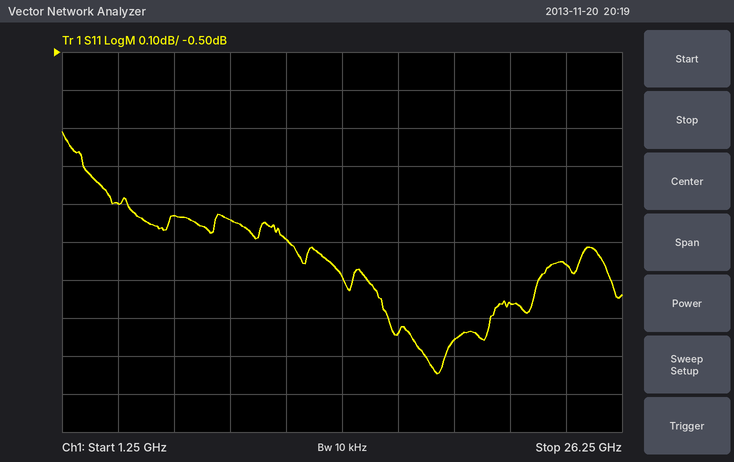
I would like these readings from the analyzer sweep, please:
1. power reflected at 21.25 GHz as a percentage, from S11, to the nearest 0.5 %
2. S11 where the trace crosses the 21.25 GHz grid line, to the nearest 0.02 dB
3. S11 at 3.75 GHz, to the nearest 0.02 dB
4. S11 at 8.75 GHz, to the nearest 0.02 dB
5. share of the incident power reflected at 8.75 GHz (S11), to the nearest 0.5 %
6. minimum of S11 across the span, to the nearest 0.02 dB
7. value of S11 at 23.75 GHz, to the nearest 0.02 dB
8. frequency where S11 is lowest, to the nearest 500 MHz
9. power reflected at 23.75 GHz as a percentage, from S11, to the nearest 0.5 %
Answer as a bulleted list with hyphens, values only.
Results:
- 76.5 %
- -1.16 dB
- -0.90 dB
- -0.94 dB
- 80.5 %
- -1.34 dB
- -1.06 dB
- 18.0 GHz
- 78.5 %
